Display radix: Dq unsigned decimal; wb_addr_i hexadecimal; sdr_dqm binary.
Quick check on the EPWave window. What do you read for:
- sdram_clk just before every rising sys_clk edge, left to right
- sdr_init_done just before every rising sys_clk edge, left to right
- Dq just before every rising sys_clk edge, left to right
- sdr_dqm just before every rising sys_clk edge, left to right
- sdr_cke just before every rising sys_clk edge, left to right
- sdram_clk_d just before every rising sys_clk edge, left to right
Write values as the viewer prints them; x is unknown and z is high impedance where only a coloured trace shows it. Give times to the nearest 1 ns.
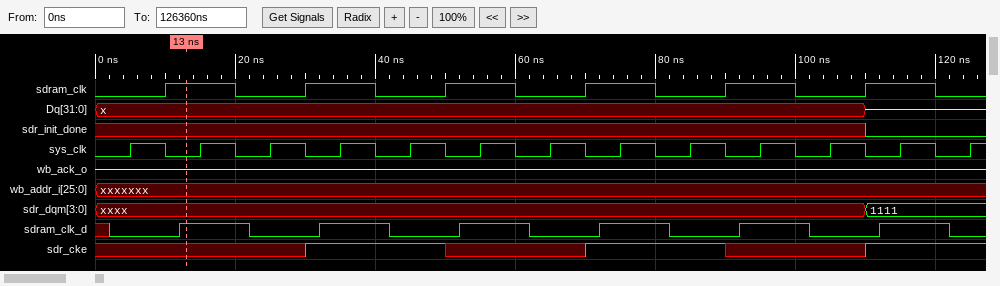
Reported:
0 1 0 1 0 1 0 1 0 1 0 1 0
x x x x x x x x x x x 0 0
x, x, x, x, x, x, x, x, x, x, x, z, z
xxxx, xxxx, xxxx, xxxx, xxxx, xxxx, xxxx, xxxx, xxxx, xxxx, xxxx, 1111, 1111
x x x 1 1 x x 1 1 x x 1 1
0 1 0 1 0 1 0 1 0 1 0 1 0
